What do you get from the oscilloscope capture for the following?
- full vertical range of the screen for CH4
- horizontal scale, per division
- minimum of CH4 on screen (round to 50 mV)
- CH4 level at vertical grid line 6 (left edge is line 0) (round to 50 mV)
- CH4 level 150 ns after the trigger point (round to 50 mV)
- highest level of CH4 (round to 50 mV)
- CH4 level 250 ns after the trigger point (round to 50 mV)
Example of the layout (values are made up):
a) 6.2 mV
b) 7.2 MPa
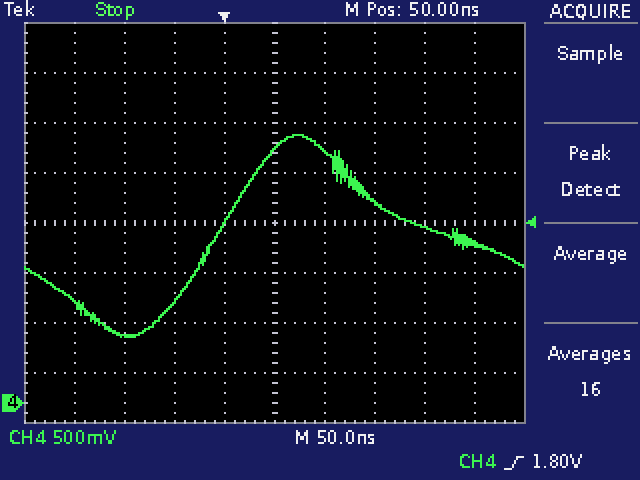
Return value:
a) 4 V
b) 50 ns
c) 650 mV
d) 2.50 V
e) 2.00 V
f) 2.70 V
g) 1.60 V
